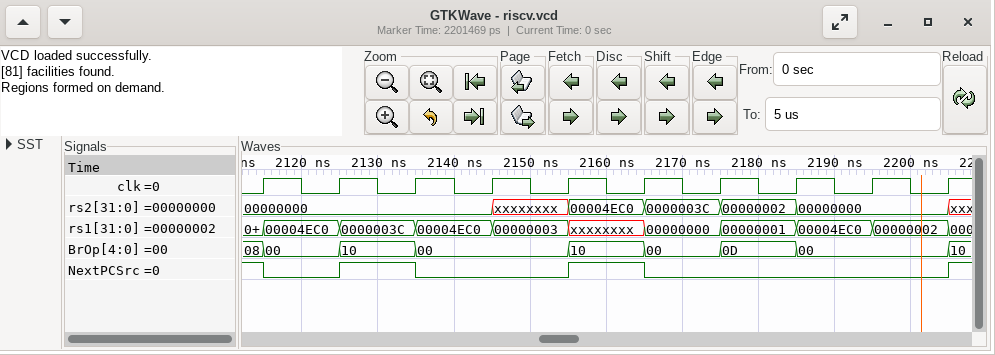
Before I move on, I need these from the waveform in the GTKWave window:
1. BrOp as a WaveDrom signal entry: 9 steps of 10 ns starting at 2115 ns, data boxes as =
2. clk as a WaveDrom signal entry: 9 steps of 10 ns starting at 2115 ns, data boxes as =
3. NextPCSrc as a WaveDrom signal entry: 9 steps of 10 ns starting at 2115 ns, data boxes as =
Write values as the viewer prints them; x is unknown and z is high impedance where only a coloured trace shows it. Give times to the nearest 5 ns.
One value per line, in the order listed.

{name: 'BrOp', wave: '===.====.', data: '00 10 00 10 00 0D 00'}
{name: 'clk', wave: 'p........'}
{name: 'NextPCSrc', wave: '010.10...'}
